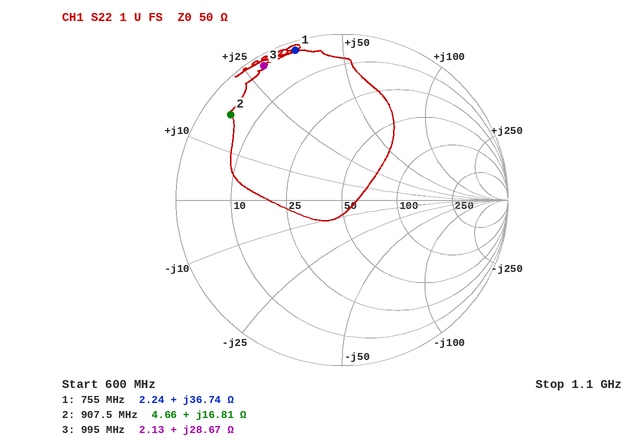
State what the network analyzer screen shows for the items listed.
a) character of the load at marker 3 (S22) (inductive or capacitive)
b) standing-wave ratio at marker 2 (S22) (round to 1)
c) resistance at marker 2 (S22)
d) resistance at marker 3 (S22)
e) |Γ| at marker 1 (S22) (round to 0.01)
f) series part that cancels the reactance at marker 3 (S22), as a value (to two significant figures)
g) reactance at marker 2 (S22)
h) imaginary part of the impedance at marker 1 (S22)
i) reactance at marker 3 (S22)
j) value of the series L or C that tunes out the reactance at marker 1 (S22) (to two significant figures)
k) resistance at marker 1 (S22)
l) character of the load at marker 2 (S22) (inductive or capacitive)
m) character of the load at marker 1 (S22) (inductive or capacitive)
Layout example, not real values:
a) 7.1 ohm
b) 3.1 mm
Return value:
a) inductive
b) 12
c) 4.66 Ω
d) 2.13 Ω
e) 0.94
f) 5.6 pF
g) +16.81 Ω
h) +36.74 Ω
i) +28.67 Ω
j) 5.7 pF
k) 2.24 Ω
l) inductive
m) inductive
